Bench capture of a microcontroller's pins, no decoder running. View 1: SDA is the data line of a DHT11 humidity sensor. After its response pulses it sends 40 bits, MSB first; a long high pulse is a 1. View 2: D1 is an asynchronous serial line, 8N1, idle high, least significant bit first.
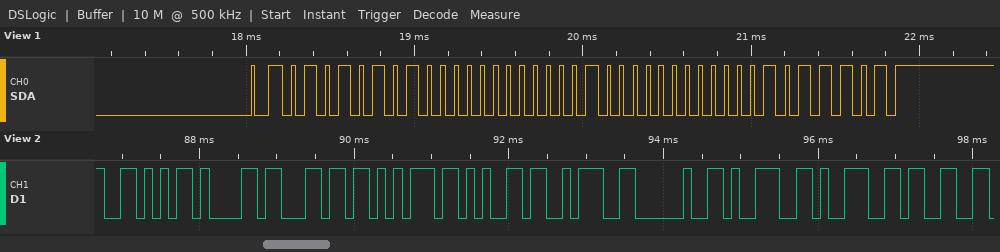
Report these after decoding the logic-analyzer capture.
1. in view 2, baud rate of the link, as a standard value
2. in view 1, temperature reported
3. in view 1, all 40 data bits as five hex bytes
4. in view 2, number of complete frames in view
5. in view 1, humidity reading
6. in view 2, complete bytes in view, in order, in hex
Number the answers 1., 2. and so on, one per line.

1. 9600 baud
2. 8.0 °C
3. 55 00 08 00 5D
4. 10
5. 85 %
6. 56 61 6C 75 65 3A 20 39 39 33
